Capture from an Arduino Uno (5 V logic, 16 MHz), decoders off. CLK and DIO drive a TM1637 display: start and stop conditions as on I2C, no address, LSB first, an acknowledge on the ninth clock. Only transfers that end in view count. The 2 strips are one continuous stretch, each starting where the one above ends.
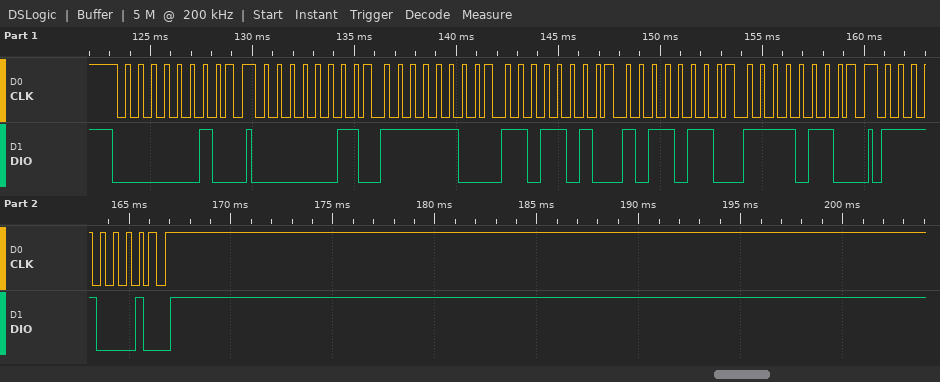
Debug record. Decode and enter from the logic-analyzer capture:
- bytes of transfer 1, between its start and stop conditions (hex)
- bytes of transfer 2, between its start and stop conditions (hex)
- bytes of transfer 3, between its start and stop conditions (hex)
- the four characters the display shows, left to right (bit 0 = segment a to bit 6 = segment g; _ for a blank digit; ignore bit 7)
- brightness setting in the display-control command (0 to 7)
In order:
40
C0 3F 5B 6D 6F
8F
0259
7
